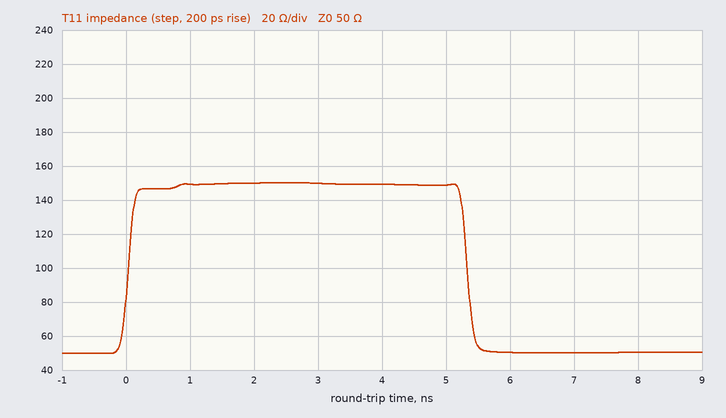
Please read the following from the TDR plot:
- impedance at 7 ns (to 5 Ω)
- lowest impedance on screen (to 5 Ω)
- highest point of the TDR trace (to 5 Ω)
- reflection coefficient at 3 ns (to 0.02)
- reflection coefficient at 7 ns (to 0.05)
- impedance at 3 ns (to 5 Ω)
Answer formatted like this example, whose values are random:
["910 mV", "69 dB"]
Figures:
["50 Ω", "50 Ω", "150 Ω", "+0.50", "0.00", "150 Ω"]
